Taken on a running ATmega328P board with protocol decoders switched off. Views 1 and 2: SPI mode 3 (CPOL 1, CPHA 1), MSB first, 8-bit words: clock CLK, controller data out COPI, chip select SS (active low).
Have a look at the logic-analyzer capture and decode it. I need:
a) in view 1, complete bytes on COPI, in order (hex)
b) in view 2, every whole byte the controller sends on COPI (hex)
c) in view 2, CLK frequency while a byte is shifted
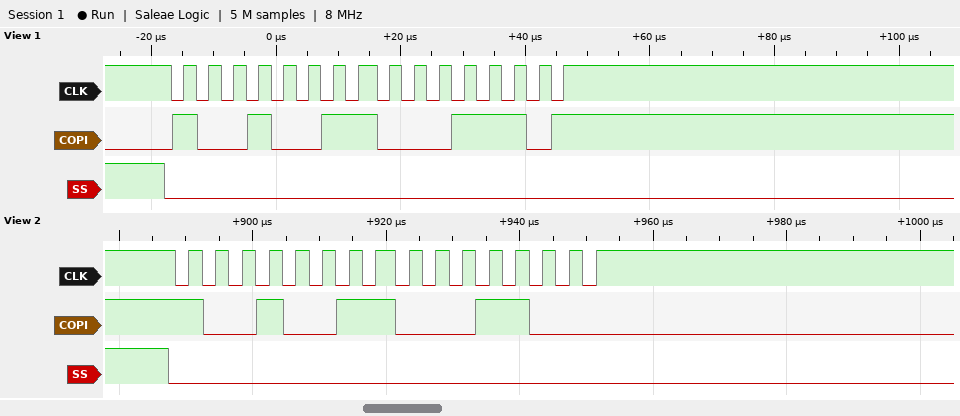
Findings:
93 1D
93 18
250 kHz
